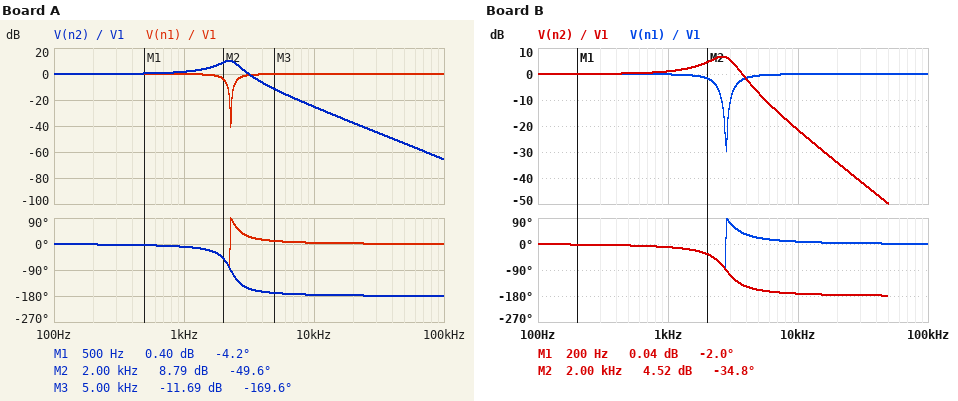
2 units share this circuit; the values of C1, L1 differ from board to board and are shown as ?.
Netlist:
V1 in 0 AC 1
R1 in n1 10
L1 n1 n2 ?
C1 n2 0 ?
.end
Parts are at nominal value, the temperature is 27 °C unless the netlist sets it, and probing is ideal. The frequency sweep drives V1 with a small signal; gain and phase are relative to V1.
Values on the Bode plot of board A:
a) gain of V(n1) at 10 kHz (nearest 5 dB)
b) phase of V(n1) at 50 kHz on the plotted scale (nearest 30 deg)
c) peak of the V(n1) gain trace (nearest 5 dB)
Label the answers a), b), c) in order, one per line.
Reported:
a) 0 dB
b) 0 deg
c) 0 dB
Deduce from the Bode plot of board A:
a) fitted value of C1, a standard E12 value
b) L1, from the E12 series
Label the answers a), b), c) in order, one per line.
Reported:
a) 2.2 µF
b) 2.2 mH
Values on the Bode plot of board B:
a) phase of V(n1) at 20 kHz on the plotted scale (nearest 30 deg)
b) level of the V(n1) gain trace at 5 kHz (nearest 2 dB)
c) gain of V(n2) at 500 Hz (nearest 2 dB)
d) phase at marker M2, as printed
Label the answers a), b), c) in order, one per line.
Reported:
a) 0 deg
b) 0 dB
c) 0 dB
d) -34.8 deg
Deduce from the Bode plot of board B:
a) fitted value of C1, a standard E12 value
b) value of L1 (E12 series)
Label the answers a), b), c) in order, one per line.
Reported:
a) 2.7 µF
b) 1.2 mH
